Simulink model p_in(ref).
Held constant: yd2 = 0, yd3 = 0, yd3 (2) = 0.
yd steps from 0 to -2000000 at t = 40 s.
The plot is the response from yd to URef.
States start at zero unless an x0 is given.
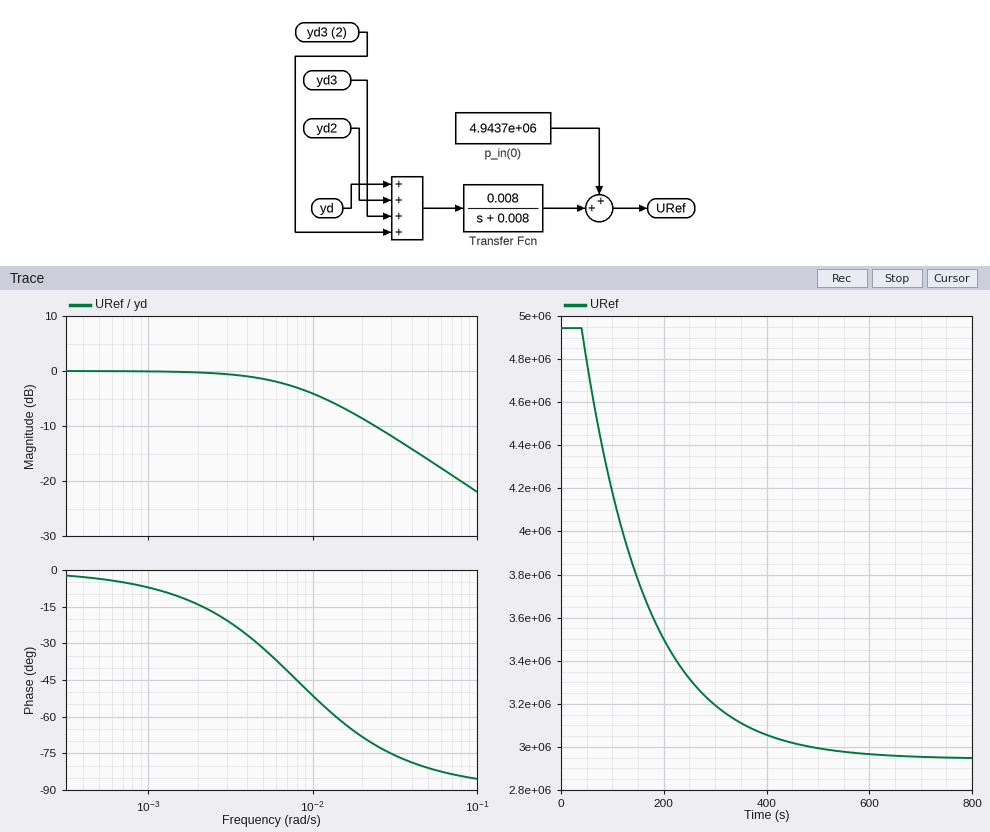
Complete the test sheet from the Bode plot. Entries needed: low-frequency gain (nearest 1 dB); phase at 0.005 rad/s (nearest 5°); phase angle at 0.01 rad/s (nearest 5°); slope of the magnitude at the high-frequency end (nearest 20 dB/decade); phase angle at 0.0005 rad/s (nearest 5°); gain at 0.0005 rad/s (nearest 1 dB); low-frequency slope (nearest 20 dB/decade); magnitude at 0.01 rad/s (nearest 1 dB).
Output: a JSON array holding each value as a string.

["0 dB", "-30°", "-50°", "-20 dB/decade", "-5°", "0 dB", "0 dB/decade", "-4 dB"]
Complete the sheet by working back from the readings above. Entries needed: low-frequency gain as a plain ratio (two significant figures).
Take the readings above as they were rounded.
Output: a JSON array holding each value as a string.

["1.0"]
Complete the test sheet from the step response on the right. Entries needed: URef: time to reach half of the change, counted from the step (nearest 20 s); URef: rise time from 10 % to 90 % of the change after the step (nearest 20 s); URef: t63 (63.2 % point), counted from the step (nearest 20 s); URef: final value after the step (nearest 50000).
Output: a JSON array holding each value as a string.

["80 s", "280 s", "120 s", "2950000"]
